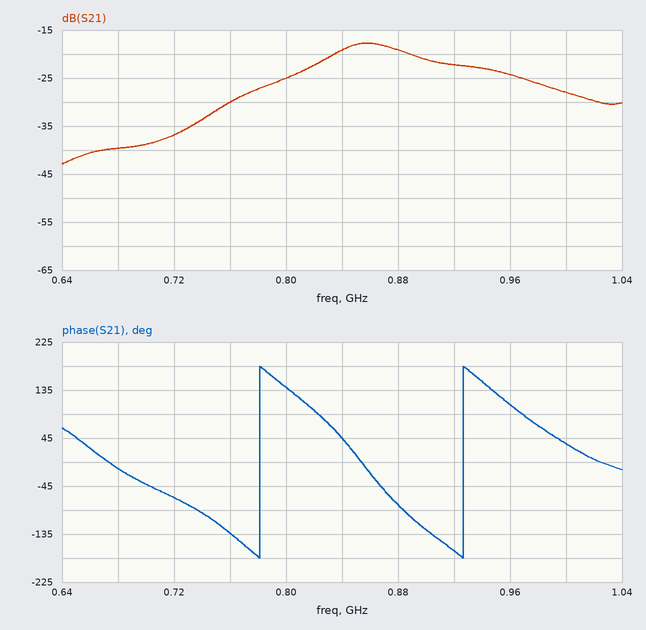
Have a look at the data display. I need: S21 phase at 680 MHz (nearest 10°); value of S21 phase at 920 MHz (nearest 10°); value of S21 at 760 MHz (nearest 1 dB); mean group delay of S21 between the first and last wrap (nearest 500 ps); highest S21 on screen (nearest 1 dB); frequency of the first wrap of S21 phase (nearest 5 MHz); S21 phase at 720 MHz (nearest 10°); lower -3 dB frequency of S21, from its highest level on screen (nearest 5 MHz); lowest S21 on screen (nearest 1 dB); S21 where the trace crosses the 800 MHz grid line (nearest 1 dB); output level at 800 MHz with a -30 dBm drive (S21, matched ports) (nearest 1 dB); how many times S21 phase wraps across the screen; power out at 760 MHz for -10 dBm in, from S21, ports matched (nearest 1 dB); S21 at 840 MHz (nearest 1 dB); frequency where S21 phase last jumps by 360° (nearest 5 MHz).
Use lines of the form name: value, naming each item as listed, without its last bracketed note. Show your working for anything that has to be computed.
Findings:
S21 phase at 680 MHz: -10°
value of S21 phase at 920 MHz: -170°
value of S21 at 760 MHz: -30 dB
mean group delay of S21 between the first and last wrap: 1 cycle / (925 MHz − 780 MHz) ≈ 6.90 ns, so 7.0 ns to the nearest 500 ps
highest S21 on screen: -18 dB
frequency of the first wrap of S21 phase: 780 MHz
S21 phase at 720 MHz: -70°
lower -3 dB frequency of S21, from its highest level on screen: 830 MHz
lowest S21 on screen: -43 dB
S21 where the trace crosses the 800 MHz grid line: -25 dB
output level at 800 MHz with a -30 dBm drive (S21, matched ports): -30 dBm + (-25 dB) = -55 dBm
how many times S21 phase wraps across the screen: 2
power out at 760 MHz for -10 dBm in, from S21, ports matched: -10 dBm + (-30 dB) = -40 dBm
S21 at 840 MHz: -19 dB
frequency where S21 phase last jumps by 360°: 925 MHz
